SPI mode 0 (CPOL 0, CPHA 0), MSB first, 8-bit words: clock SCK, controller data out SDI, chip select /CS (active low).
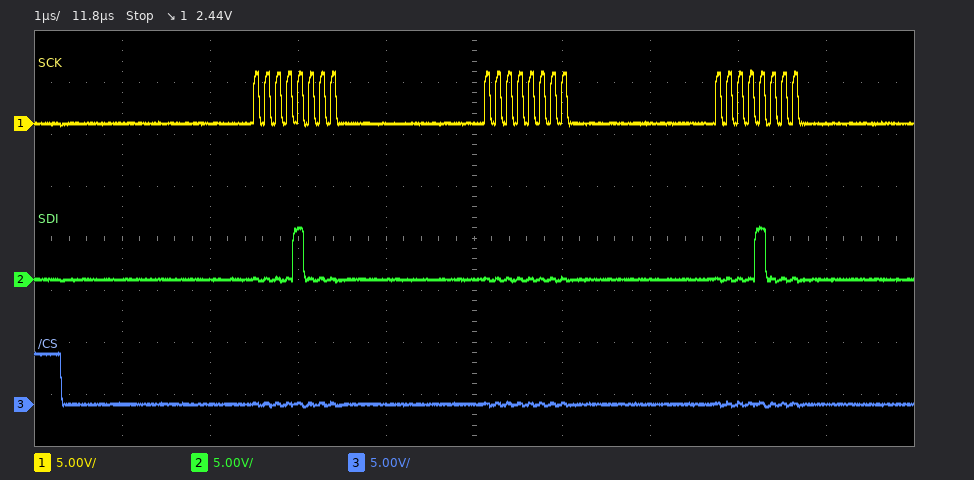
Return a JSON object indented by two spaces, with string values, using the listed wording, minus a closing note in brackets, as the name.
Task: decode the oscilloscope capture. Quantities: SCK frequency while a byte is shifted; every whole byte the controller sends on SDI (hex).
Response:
{
  "SCK frequency while a byte is shifted": "8 MHz",
  "every whole byte the controller sends on SDI": "08 00 08"
}
